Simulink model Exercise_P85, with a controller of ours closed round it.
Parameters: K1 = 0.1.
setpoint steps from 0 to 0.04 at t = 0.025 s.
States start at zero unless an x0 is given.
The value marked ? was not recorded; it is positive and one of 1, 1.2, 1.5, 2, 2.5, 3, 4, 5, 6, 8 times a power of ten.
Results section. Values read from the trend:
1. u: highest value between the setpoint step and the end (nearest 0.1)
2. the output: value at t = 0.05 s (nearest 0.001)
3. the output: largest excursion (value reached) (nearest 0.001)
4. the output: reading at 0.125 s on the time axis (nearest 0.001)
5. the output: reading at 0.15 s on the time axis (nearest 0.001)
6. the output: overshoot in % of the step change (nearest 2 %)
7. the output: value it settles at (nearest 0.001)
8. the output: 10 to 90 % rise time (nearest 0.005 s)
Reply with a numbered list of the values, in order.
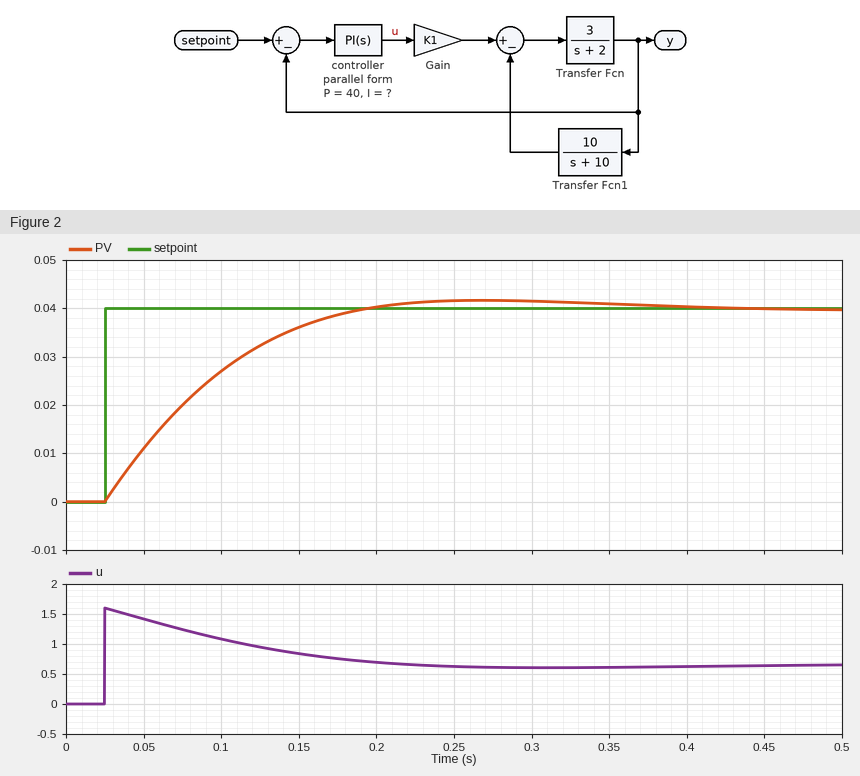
1. 1.6
2. 0.011
3. 0.042
4. 0.032
5. 0.036
6. 4 %
7. 0.040
8. 0.115 s
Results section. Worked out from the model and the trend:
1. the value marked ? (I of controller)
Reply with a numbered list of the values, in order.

1. 300
